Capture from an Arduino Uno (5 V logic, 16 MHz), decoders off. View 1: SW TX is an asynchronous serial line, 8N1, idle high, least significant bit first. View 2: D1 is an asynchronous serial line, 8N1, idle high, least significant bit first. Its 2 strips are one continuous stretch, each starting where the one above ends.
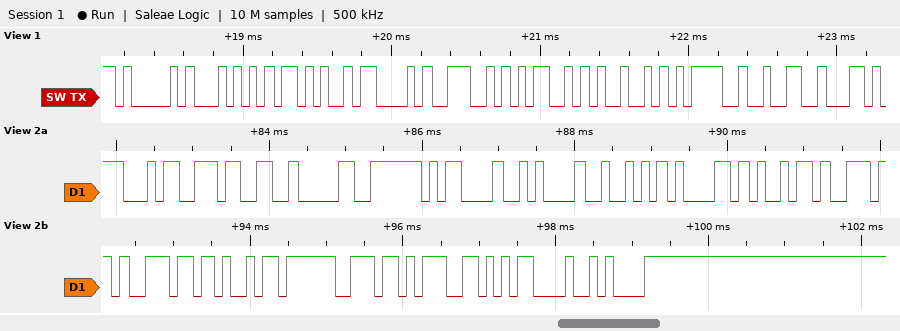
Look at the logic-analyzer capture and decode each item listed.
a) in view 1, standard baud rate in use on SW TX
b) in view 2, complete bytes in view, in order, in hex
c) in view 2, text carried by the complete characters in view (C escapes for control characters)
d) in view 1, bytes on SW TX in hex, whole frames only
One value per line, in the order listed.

19200 baud
34 33 30 0D 0A 52 61 69 6E 6E 69 6E 67 0D 0A
"430\r\nRainning\r\n"
41 54 2B 43 4E 4D 49 3D 32
